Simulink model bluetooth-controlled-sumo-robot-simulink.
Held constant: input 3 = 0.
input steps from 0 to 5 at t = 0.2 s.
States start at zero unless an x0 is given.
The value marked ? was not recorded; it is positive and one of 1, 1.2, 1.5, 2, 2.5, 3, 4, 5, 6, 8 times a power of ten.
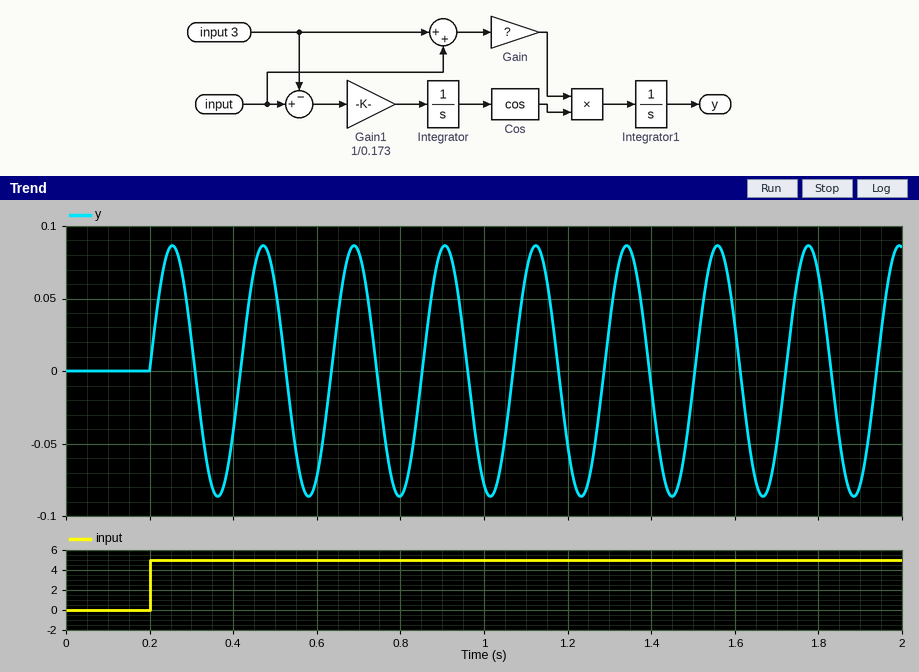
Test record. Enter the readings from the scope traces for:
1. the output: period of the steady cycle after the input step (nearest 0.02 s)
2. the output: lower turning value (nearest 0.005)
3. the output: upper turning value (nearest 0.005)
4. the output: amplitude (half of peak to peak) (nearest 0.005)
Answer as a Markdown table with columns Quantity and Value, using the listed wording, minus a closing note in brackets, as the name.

| Quantity | Value |
|---|---|
| the output: period of the steady cycle after the input step | 0.22 s |
| the output: lower turning value | -0.085 |
| the output: upper turning value | 0.085 |
| the output: amplitude (half of peak to peak) | 0.085 |
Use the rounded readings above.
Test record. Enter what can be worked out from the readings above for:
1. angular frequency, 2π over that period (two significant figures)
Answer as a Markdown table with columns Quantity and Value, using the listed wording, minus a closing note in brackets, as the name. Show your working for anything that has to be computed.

| Quantity | Value |
|---|---|
| angular frequency, 2π over that period | 2π / 0.22 = 29 rad/s |
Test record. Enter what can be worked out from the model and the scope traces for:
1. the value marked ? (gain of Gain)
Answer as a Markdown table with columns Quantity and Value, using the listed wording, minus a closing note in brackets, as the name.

| Quantity | Value |
|---|---|
| the value marked ? | 0.5 |
